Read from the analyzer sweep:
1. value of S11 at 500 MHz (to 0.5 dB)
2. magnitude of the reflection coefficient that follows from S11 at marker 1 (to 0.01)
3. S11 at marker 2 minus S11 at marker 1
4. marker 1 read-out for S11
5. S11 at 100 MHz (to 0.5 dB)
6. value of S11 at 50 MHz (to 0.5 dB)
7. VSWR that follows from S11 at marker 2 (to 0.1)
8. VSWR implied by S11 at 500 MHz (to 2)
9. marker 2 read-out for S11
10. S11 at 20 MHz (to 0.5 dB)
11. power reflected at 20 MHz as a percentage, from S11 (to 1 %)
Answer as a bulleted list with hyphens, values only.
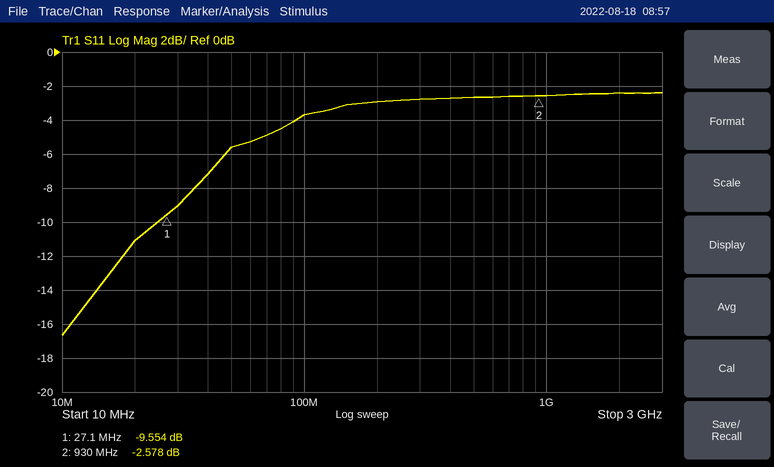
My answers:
- -2.5 dB
- 0.33
- 6.976 dB
- -9.554 dB
- -3.5 dB
- -5.5 dB
- 6.8
- 6
- -2.578 dB
- -11.0 dB
- 8 %
